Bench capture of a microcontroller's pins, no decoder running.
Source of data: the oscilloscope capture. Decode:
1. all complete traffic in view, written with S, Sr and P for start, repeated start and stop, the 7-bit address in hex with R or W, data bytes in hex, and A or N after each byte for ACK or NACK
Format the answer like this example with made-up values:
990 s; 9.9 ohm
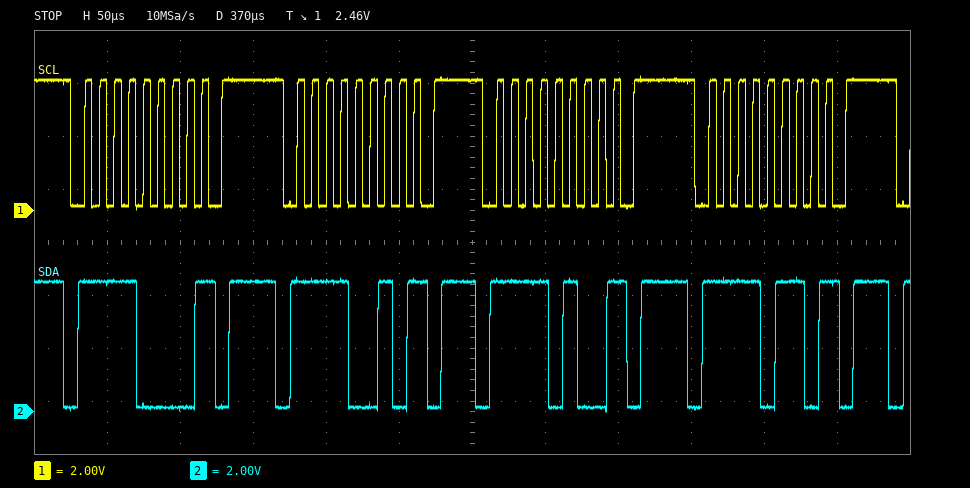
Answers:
S 78W N P S 79W N P S 7AW N P S 7BW N P
